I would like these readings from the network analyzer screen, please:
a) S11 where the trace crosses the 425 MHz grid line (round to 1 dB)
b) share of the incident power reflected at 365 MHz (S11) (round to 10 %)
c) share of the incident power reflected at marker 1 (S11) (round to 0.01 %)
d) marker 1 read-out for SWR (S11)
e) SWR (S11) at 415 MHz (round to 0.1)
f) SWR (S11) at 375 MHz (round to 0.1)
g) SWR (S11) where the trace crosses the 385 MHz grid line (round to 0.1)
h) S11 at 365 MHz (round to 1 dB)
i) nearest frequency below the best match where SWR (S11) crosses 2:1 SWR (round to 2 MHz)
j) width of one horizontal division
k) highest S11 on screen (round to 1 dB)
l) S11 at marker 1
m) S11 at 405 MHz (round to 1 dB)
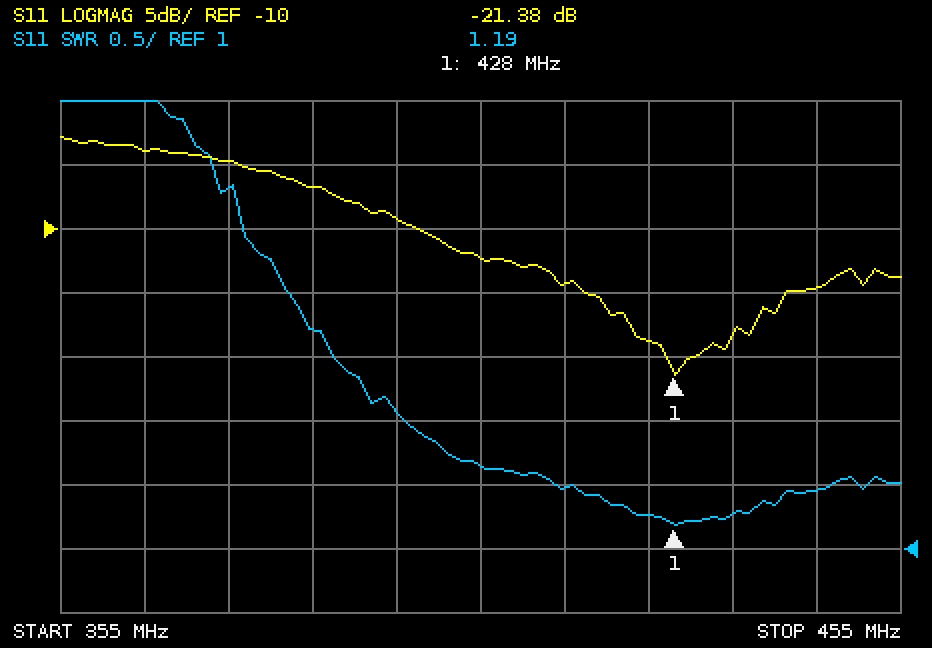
-19 dB
40 %
0.73 %
1.19
1.5
3.8
2.7
-4 dB
396 MHz
10 MHz
-3 dB
-21.38 dB
-12 dB
